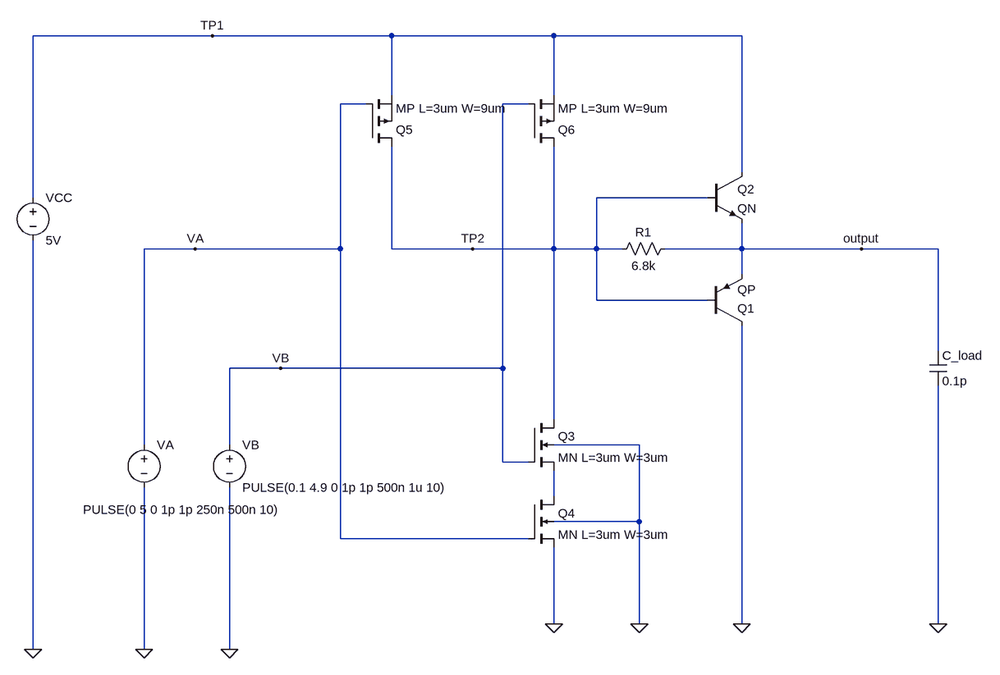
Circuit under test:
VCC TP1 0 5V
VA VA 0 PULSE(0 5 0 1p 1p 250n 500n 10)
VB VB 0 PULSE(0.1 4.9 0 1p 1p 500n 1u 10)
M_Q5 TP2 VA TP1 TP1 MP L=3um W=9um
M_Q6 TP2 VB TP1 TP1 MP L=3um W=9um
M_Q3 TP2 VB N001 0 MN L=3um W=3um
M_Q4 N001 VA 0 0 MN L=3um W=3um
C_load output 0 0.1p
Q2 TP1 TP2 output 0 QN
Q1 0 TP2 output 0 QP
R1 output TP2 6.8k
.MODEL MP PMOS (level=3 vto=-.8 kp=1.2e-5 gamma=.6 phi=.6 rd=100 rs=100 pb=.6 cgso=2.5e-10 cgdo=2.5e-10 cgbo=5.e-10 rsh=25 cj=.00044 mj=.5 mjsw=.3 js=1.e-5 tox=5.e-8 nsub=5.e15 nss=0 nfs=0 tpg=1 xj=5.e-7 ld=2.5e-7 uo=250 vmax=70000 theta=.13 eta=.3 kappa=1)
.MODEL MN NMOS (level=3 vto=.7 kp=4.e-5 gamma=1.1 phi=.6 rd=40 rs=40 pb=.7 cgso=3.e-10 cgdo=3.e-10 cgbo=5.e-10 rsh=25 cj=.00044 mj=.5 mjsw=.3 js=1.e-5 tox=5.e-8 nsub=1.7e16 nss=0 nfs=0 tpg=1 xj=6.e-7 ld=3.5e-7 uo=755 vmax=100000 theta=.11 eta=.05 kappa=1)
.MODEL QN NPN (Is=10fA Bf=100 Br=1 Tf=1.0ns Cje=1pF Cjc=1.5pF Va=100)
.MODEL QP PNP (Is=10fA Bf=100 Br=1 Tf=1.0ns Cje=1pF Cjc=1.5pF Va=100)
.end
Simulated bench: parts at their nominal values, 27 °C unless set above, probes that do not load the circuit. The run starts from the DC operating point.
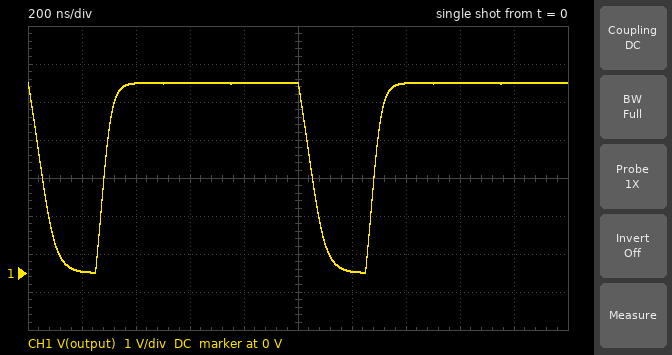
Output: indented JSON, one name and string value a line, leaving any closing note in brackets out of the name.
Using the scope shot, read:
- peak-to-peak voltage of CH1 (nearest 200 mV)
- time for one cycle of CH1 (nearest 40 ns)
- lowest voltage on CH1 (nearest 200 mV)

{
  "peak-to-peak voltage of CH1": "5.0 V",
  "time for one cycle of CH1": "1.00 µs",
  "lowest voltage on CH1": "0 V"
}
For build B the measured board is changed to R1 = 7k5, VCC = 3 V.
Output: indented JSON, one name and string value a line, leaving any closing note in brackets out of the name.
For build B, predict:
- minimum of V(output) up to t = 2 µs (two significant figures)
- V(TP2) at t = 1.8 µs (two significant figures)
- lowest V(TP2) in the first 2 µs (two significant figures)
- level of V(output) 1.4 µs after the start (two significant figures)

{
  "minimum of V(output) up to t = 2 µs": "-1.3 mV",
  "V(TP2) at t = 1.8 µs": "3.0 V",
  "lowest V(TP2) in the first 2 µs": "-1.7 mV",
  "level of V(output) 1.4 µs after the start": "2.9 V"
}
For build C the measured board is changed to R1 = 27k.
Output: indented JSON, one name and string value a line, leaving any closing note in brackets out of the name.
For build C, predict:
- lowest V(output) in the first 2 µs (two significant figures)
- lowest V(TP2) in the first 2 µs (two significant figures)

{
  "lowest V(output) in the first 2 µs": "14 mV",
  "lowest V(TP2) in the first 2 µs": "2.3 mV"
}
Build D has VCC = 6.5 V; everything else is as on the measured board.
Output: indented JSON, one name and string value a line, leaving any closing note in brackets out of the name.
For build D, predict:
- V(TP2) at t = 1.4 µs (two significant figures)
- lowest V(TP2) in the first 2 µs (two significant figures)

{
  "V(TP2) at t = 1.4 µs": "6.5 V",
  "lowest V(TP2) in the first 2 µs": "440 mV"
}
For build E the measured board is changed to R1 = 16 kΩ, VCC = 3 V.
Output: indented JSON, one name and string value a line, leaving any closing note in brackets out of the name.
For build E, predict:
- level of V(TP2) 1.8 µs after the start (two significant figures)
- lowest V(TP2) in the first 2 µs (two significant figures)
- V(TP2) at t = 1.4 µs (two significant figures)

{
  "level of V(TP2) 1.8 µs after the start": "3.0 V",
  "lowest V(TP2) in the first 2 µs": "-1.6 mV",
  "V(TP2) at t = 1.4 µs": "2.9 V"
}
